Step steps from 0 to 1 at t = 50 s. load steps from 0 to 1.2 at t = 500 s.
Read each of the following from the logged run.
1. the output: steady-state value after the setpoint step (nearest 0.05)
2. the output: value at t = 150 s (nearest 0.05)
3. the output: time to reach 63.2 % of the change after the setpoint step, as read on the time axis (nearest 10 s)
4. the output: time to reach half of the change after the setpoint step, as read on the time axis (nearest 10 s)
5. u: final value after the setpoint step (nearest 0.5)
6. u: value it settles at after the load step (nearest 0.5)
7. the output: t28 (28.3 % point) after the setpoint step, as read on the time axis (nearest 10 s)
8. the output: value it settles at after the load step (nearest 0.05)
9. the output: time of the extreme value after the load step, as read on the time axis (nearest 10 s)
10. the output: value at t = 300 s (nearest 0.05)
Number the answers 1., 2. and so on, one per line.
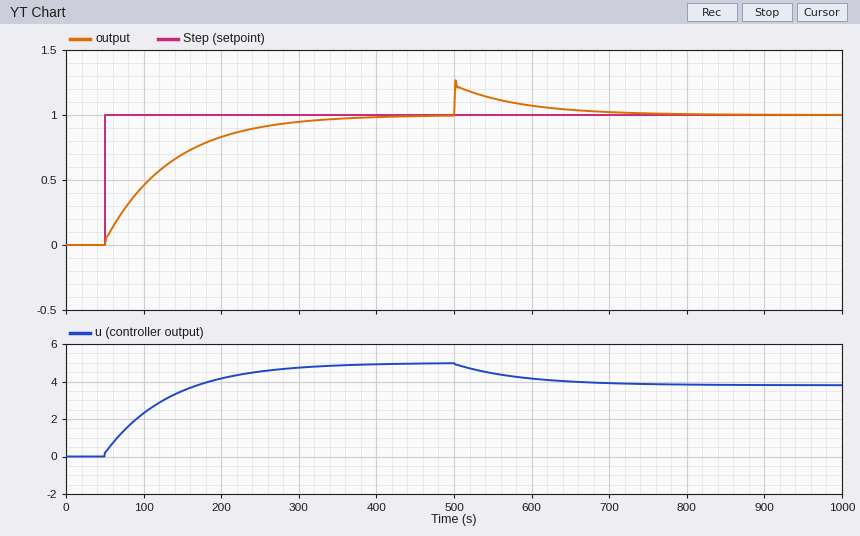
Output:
1. 1.00
2. 0.70
3. 130 s
4. 110 s
5. 5.0
6. 4.0
7. 80 s
8. 1.00
9. 500 s
10. 0.95
